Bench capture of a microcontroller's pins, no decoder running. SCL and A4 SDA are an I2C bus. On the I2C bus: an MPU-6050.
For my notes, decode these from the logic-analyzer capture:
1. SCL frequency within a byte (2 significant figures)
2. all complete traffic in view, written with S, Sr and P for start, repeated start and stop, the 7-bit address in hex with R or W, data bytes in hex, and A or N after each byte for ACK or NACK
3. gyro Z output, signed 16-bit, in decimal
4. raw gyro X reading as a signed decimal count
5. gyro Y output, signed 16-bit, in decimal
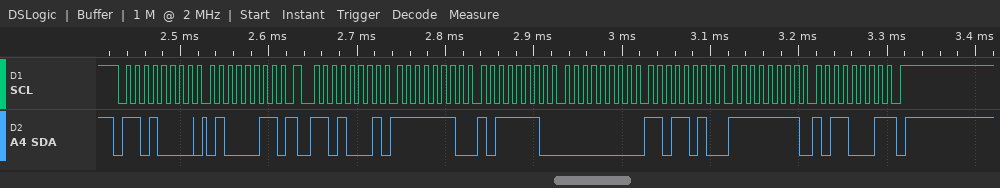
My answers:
100 kHz
S 68W A 43 A Sr 68R A FE A BE A 00 A DA A FF A B1 N P
-79
-322
218
